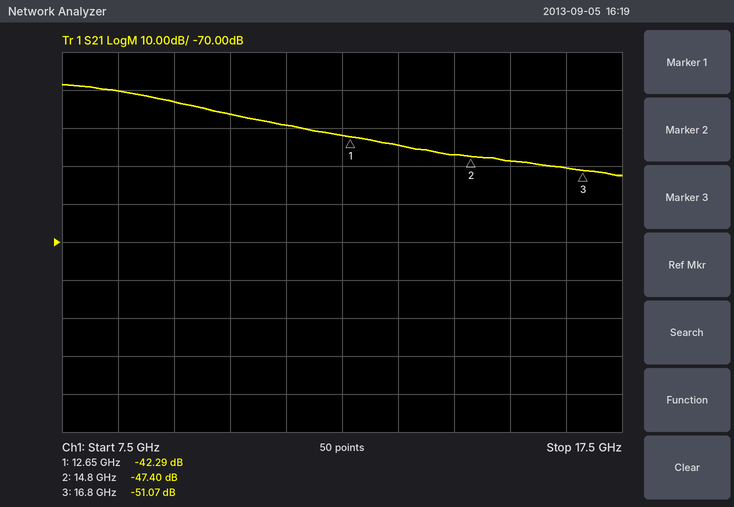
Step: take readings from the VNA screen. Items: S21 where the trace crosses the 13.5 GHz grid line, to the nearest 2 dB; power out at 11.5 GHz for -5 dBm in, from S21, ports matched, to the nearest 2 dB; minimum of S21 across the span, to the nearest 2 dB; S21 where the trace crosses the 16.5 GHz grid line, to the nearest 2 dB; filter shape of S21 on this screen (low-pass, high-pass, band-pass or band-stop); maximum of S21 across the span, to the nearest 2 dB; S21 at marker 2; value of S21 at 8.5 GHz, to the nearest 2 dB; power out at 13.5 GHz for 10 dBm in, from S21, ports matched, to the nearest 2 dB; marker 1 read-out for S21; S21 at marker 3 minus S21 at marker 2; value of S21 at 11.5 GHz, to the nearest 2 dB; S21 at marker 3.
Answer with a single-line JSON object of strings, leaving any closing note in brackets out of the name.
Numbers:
{"S21 where the trace crosses the 13.5 GHz grid line, to the nearest 2 dB": "-44 dB", "power out at 11.5 GHz for -5 dBm in, from S21, ports matched, to the nearest 2 dB": "-44 dBm", "minimum of S21 across the span, to the nearest 2 dB": "-52 dB", "S21 where the trace crosses the 16.5 GHz grid line, to the nearest 2 dB": "-50 dB", "filter shape of S21 on this screen": "low-pass", "maximum of S21 across the span, to the nearest 2 dB": "-28 dB", "S21 at marker 2": "-47.40 dB", "value of S21 at 8.5 GHz, to the nearest 2 dB": "-30 dB", "power out at 13.5 GHz for 10 dBm in, from S21, ports matched, to the nearest 2 dB": "-34 dBm", "marker 1 read-out for S21": "-42.29 dB", "S21 at marker 3 minus S21 at marker 2": "-3.67 dB", "value of S21 at 11.5 GHz, to the nearest 2 dB": "-40 dB", "S21 at marker 3": "-51.07 dB"}
